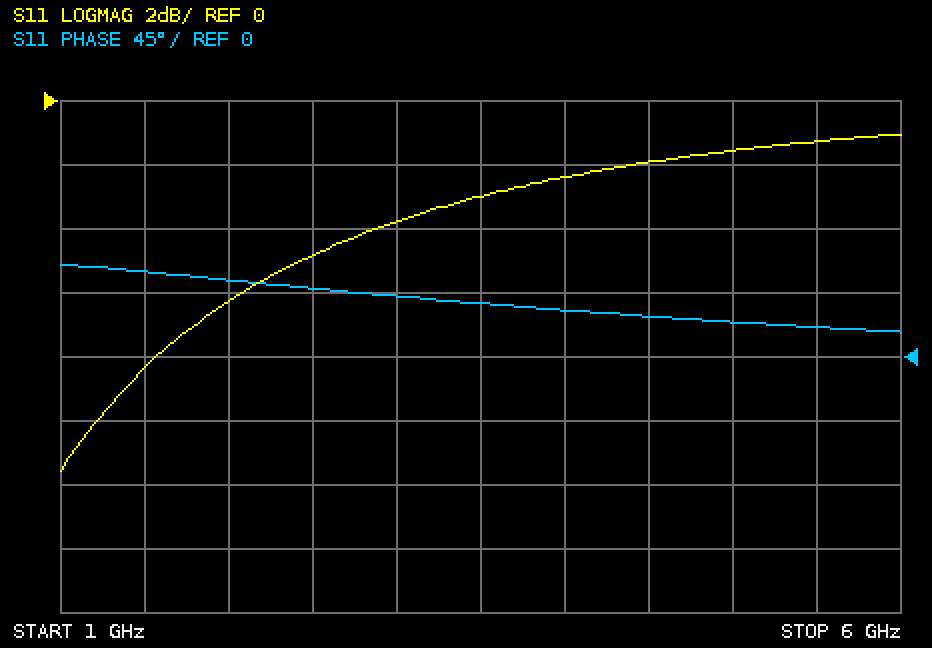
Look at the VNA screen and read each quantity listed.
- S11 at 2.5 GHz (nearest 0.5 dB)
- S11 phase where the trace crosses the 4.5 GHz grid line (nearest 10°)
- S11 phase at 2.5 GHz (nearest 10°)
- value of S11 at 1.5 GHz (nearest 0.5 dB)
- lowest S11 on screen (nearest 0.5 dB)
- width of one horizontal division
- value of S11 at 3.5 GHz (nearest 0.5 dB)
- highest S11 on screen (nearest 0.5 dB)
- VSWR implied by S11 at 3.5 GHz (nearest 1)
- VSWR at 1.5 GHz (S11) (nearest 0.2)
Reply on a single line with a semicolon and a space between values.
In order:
-5.0 dB; 30°; 50°; -8.5 dB; -11.5 dB; 500 MHz; -3.0 dB; -1.0 dB; 6; 2.2
